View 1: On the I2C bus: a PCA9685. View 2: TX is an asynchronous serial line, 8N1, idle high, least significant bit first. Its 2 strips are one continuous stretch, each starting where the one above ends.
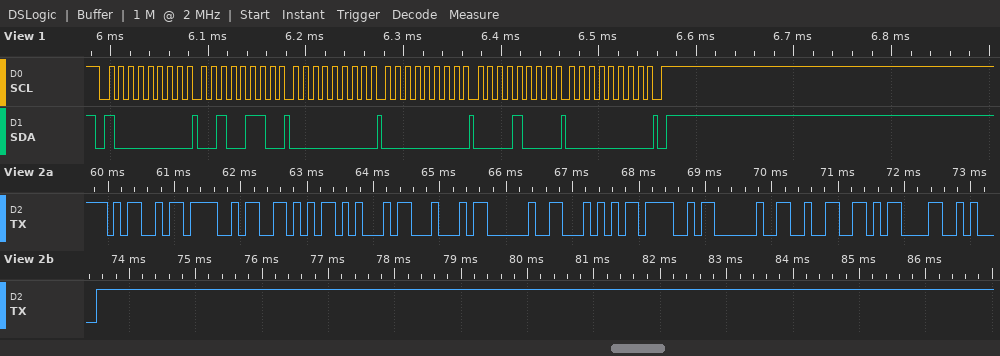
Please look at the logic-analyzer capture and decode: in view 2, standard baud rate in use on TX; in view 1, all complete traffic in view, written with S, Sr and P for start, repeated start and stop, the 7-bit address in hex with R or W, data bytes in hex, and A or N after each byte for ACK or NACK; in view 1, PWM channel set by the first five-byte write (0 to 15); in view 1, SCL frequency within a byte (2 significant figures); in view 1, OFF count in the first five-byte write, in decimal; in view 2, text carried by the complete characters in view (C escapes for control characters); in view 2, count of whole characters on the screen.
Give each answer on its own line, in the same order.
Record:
9600 baud
S 40W A 26 A 00 A 00 A 08 A 00 A P
8
100 kHz
8
"MOVED TO 2\r\n"
12
